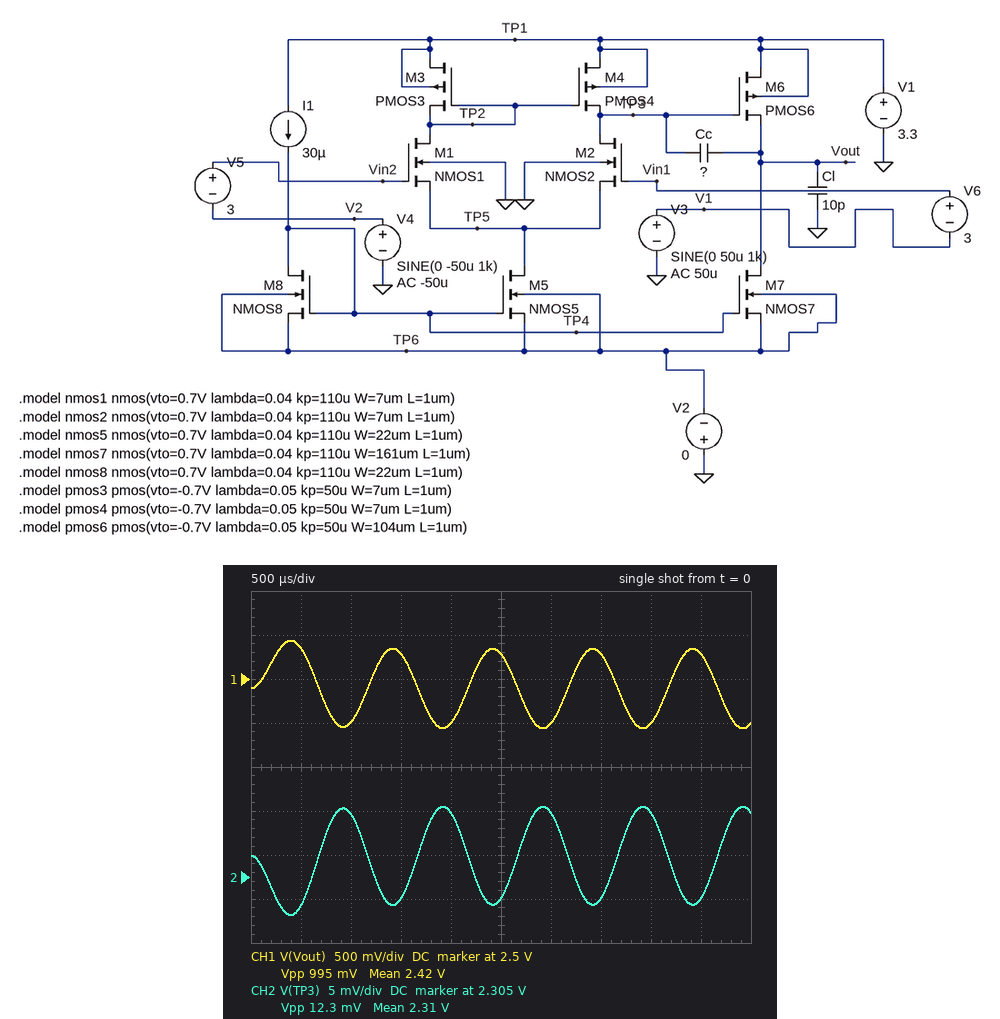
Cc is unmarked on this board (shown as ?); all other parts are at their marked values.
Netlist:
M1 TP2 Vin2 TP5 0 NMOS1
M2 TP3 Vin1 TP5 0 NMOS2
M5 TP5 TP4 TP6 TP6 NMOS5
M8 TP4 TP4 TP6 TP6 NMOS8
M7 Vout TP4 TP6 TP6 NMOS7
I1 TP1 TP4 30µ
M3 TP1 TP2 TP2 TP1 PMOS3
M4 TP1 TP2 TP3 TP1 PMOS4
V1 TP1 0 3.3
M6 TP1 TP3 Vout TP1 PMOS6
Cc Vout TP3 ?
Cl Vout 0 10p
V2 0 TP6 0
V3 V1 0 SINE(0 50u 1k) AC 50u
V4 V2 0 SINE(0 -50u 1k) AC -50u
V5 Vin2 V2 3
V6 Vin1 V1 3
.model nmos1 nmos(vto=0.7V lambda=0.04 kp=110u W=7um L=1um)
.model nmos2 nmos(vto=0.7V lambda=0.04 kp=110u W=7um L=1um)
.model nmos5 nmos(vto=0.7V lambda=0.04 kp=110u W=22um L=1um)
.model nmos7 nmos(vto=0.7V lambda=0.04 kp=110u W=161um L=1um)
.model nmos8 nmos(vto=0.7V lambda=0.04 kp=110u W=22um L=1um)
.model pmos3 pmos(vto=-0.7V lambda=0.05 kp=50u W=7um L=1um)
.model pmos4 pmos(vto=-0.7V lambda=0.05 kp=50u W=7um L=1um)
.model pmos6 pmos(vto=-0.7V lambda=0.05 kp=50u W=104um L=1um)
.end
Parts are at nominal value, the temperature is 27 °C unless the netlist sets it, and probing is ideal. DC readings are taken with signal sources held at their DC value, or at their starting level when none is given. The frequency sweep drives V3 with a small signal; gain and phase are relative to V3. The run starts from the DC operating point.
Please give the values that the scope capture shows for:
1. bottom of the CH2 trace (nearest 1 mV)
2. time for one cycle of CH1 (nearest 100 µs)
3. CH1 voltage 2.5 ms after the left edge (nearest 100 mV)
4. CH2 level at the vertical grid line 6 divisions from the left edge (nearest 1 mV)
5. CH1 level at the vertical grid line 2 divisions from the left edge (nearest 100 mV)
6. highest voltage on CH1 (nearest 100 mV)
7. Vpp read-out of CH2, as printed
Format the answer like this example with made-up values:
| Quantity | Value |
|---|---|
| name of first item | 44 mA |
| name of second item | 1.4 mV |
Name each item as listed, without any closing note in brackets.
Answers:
| Quantity | Value |
|---|---|
| bottom of the CH2 trace | 2.301 V |
| time for one cycle of CH1 | 1.0 ms |
| CH1 voltage 2.5 ms after the left edge | 2.8 V |
| CH2 level at the vertical grid line 6 divisions from the left edge | 2.312 V |
| CH1 level at the vertical grid line 2 divisions from the left edge | 2.0 V |
| highest voltage on CH1 | 2.9 V |
| Vpp read-out of CH2, as printed | 12.3 mV |
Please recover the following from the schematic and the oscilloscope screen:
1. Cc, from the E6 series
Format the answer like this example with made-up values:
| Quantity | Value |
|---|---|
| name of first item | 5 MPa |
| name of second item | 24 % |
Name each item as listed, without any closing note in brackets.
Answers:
| Quantity | Value |
|---|---|
| Cc, from the E6 series | 4.7 pF |
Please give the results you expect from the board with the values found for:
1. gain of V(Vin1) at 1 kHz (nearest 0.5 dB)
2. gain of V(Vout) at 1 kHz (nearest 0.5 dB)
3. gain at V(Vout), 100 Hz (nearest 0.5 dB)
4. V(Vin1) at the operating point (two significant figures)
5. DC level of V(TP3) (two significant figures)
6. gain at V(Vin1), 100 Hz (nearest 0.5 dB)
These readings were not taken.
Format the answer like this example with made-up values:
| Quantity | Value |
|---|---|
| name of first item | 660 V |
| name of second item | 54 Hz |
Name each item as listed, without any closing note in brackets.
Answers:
| Quantity | Value |
|---|---|
| gain of V(Vin1) at 1 kHz | 0 dB |
| gain of V(Vout) at 1 kHz | 73.0 dB |
| gain at V(Vout), 100 Hz | 79.0 dB |
| V(Vin1) at the operating point | 3.0 V |
| DC level of V(TP3) | 2.3 V |
| gain at V(Vin1), 100 Hz | 0 dB |
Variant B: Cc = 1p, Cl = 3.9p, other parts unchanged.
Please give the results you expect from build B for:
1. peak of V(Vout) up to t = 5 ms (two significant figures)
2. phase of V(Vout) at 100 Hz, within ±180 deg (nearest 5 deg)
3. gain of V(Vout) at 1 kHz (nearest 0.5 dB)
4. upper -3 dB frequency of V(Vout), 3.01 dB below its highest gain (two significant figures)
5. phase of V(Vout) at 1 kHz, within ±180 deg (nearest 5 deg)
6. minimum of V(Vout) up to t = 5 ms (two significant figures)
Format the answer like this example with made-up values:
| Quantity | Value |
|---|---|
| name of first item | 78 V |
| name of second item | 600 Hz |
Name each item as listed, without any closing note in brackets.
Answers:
| Quantity | Value |
|---|---|
| peak of V(Vout) up to t = 5 ms | 3.0 V |
| phase of V(Vout) at 100 Hz, within ±180 deg | 0 deg |
| gain of V(Vout) at 1 kHz | 78.5 dB |
| upper -3 dB frequency of V(Vout), 3.01 dB below its highest gain | 2.6 kHz |
| phase of V(Vout) at 1 kHz, within ±180 deg | -20 deg |
| minimum of V(Vout) up to t = 5 ms | 1.5 V |
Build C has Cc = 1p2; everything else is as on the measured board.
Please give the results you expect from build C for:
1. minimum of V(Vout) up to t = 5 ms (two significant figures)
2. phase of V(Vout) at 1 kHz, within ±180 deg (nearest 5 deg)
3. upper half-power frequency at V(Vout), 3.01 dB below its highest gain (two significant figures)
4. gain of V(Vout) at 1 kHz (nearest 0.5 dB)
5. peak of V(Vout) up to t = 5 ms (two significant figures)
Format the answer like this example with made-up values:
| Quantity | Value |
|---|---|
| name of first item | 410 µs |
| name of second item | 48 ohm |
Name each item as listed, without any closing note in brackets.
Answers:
| Quantity | Value |
|---|---|
| minimum of V(Vout) up to t = 5 ms | 1.5 V |
| phase of V(Vout) at 1 kHz, within ±180 deg | -25 deg |
| upper half-power frequency at V(Vout), 3.01 dB below its highest gain | 2.2 kHz |
| gain of V(Vout) at 1 kHz | 78.5 dB |
| peak of V(Vout) up to t = 5 ms | 3.0 V |
